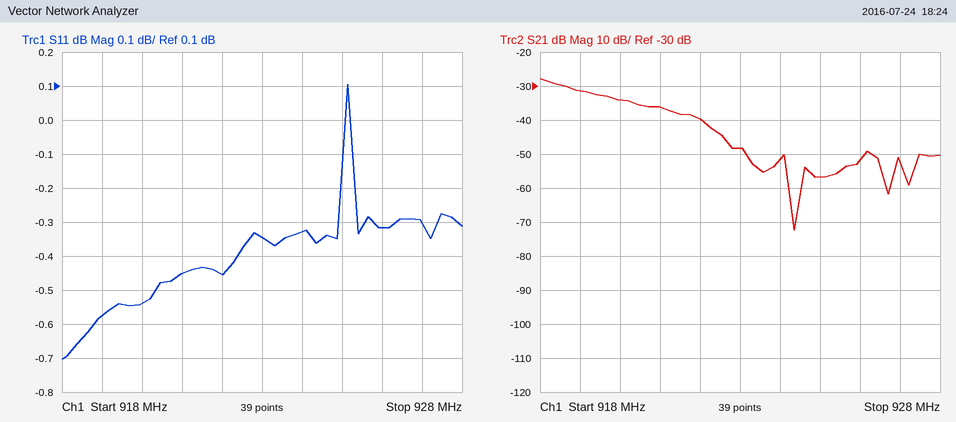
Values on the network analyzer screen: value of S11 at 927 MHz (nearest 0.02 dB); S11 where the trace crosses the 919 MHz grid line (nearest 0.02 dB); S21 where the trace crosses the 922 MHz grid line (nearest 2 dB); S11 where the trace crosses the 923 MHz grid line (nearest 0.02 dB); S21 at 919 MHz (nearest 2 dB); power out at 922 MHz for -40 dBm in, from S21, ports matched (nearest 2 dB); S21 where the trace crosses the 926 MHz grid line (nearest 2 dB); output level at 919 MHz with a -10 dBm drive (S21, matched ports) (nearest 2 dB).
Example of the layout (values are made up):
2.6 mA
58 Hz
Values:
-0.30 dB
-0.58 dB
-40 dB
-0.34 dB
-32 dB
-80 dBm
-52 dB
-42 dBm
